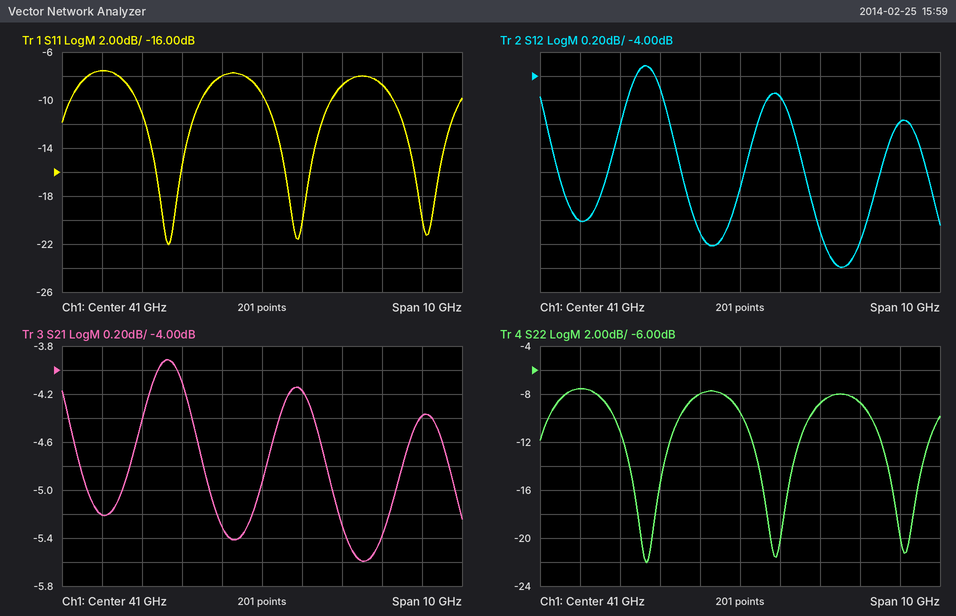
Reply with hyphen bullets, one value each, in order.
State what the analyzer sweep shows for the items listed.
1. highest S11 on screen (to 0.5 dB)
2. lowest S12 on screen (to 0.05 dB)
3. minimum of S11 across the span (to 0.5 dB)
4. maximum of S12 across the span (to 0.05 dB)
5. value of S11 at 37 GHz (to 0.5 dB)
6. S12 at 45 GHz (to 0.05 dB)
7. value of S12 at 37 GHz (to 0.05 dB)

- -7.5 dB
- -5.60 dB
- -22.0 dB
- -3.90 dB
- -7.5 dB
- -4.40 dB
- -5.20 dB
